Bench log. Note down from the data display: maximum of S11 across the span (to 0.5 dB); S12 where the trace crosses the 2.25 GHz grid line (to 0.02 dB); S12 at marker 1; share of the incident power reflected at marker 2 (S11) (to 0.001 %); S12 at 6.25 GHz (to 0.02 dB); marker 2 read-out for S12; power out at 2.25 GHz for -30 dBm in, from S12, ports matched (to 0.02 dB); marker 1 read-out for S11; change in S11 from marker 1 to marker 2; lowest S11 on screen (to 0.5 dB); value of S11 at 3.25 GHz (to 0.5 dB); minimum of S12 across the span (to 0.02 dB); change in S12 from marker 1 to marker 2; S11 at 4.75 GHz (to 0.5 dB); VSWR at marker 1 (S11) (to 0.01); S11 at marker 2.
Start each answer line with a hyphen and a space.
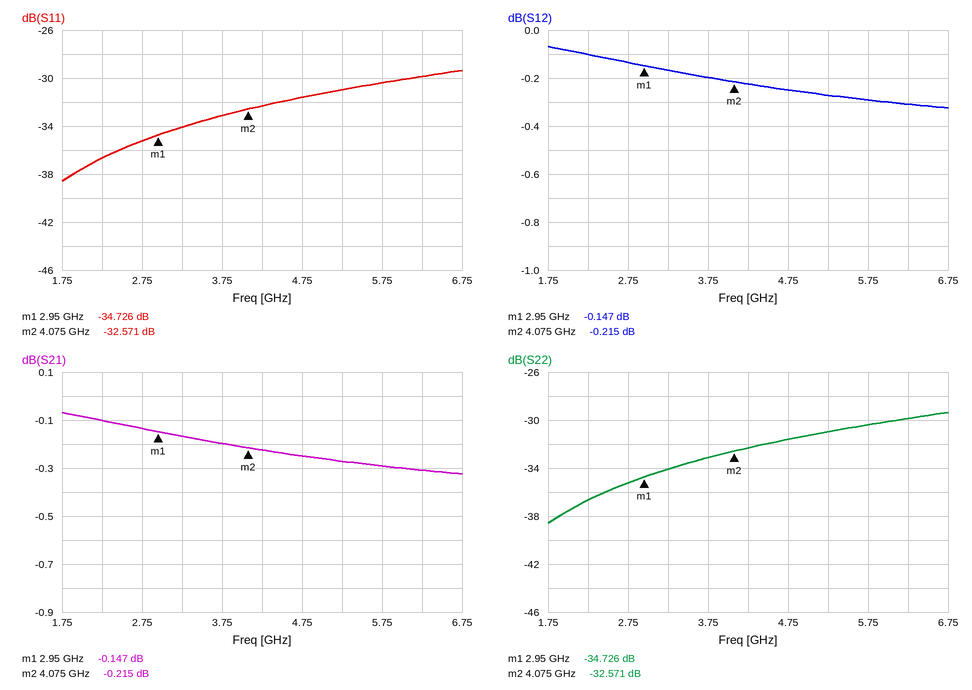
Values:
- -29.5 dB
- -0.10 dB
- -0.147 dB
- 0.055 %
- -0.30 dB
- -0.215 dB
- -30.10 dBm
- -34.726 dB
- 2.155 dB
- -38.5 dB
- -34.0 dB
- -0.32 dB
- -0.068 dB
- -31.5 dB
- 1.04
- -32.571 dB
